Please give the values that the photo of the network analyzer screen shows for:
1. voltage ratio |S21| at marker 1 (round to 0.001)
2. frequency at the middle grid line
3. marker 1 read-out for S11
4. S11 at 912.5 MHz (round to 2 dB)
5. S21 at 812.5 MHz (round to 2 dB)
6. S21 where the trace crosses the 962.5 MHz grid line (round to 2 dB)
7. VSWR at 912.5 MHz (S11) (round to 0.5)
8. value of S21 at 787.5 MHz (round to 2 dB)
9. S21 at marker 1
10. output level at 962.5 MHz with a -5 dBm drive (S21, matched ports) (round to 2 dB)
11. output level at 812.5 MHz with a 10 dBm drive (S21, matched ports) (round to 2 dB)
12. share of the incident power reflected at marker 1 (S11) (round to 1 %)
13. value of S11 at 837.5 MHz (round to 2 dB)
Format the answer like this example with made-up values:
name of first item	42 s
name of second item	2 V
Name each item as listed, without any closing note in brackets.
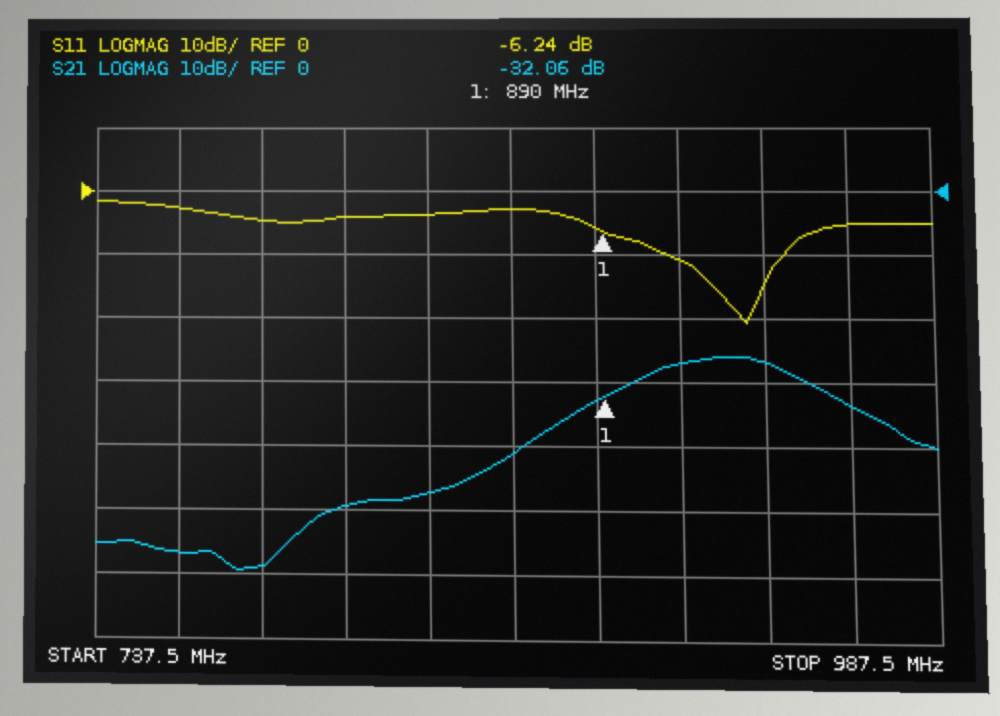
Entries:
voltage ratio |S21| at marker 1	0.025
frequency at the middle grid line	862.5 MHz
marker 1 read-out for S11	-6.24 dB
S11 at 912.5 MHz	-10 dB
S21 at 812.5 MHz	-50 dB
S21 where the trace crosses the 962.5 MHz grid line	-34 dB
VSWR at 912.5 MHz (S11)	2.0
value of S21 at 787.5 MHz	-58 dB
S21 at marker 1	-32.06 dB
output level at 962.5 MHz with a -5 dBm drive (S21, matched ports)	-38 dBm
output level at 812.5 MHz with a 10 dBm drive (S21, matched ports)	-40 dBm
share of the incident power reflected at marker 1 (S11)	24 %
value of S11 at 837.5 MHz	-4 dB
